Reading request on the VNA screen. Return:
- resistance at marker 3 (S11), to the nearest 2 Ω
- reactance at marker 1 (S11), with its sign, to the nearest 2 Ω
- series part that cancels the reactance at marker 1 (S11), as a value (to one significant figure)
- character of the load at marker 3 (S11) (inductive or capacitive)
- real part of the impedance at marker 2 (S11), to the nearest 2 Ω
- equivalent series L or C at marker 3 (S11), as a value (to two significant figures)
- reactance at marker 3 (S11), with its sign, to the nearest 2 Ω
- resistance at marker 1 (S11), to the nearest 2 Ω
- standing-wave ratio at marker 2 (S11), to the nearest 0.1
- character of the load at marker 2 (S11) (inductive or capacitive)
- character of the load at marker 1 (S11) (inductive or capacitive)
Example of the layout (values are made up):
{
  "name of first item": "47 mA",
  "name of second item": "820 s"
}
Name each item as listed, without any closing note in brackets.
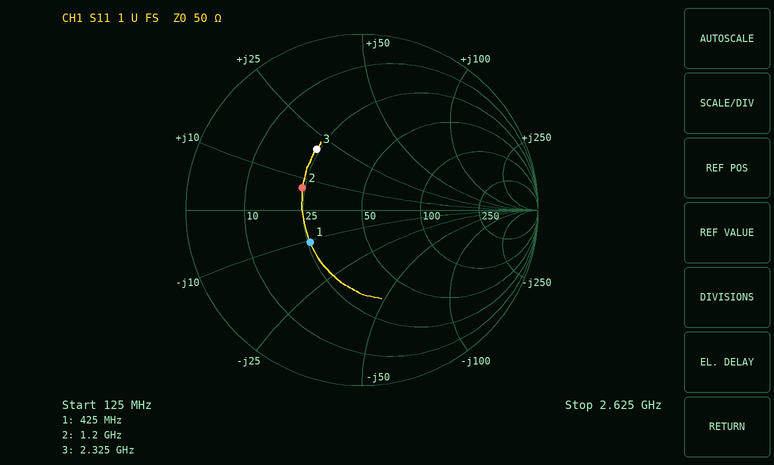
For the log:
{
  "resistance at marker 3 (S11), to the nearest 2 Ω": "24 Ω",
  "reactance at marker 1 (S11), with its sign, to the nearest 2 Ω": "-10 Ω",
  "series part that cancels the reactance at marker 1 (S11), as a value": "4 nH",
  "character of the load at marker 3 (S11)": "inductive",
  "real part of the impedance at marker 2 (S11), to the nearest 2 Ω": "24 Ω",
  "equivalent series L or C at marker 3 (S11), as a value": "1.4 nH",
  "reactance at marker 3 (S11), with its sign, to the nearest 2 Ω": "+20 Ω",
  "resistance at marker 1 (S11), to the nearest 2 Ω": "26 Ω",
  "standing-wave ratio at marker 2 (S11), to the nearest 0.1": "2.1",
  "character of the load at marker 2 (S11)": "inductive",
  "character of the load at marker 1 (S11)": "capacitive"
}
